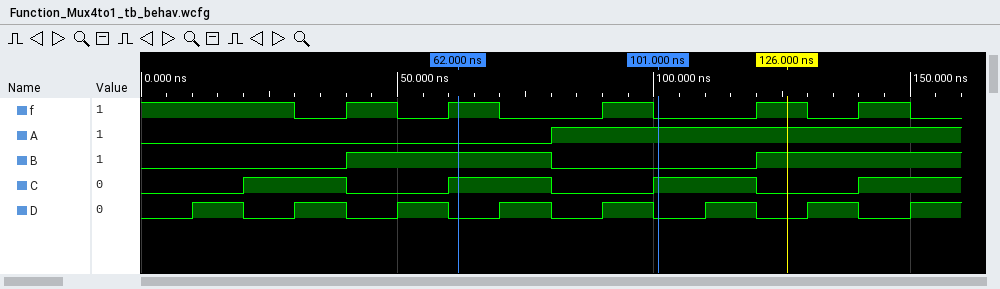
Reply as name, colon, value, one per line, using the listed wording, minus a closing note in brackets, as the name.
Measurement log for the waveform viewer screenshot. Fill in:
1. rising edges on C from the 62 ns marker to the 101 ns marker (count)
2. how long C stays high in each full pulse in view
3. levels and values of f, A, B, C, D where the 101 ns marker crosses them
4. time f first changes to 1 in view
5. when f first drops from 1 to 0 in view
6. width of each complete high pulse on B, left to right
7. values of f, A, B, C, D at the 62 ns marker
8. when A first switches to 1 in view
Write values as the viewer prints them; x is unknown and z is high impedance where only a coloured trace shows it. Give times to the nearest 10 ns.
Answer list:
rising edges on C from the 62 ns marker to the 101 ns marker: 1
how long C stays high in each full pulse in view: 20 ns, 20 ns, 20 ns
levels and values of f, A, B, C, D where the 101 ns marker crosses them: f=0, A=1, B=0, C=1, D=0
time f first changes to 1 in view: 40 ns
when f first drops from 1 to 0 in view: 30 ns
width of each complete high pulse on B, left to right: 40 ns
values of f, A, B, C, D at the 62 ns marker: f=1, A=0, B=1, C=1, D=0
when A first switches to 1 in view: 80 ns
